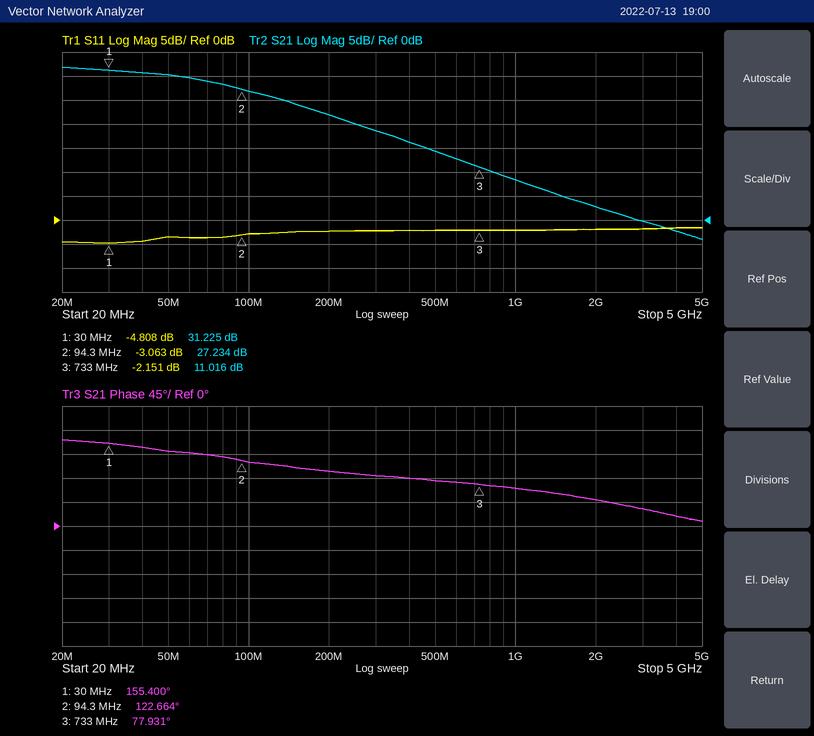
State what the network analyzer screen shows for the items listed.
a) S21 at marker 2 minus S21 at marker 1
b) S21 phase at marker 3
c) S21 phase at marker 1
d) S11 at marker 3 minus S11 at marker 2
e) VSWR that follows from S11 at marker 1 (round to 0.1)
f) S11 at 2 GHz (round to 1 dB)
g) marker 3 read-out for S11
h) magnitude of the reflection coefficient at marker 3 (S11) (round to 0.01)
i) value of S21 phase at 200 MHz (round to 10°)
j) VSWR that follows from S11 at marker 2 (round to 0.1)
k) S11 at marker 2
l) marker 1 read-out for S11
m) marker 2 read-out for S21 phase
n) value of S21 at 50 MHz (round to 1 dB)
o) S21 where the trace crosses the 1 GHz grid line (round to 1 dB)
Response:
-3.991 dB
77.931°
155.400°
0.912 dB
3.7
-2 dB
-2.151 dB
0.78
100°
5.7
-3.063 dB
-4.808 dB
122.664°
30 dB
8 dB
